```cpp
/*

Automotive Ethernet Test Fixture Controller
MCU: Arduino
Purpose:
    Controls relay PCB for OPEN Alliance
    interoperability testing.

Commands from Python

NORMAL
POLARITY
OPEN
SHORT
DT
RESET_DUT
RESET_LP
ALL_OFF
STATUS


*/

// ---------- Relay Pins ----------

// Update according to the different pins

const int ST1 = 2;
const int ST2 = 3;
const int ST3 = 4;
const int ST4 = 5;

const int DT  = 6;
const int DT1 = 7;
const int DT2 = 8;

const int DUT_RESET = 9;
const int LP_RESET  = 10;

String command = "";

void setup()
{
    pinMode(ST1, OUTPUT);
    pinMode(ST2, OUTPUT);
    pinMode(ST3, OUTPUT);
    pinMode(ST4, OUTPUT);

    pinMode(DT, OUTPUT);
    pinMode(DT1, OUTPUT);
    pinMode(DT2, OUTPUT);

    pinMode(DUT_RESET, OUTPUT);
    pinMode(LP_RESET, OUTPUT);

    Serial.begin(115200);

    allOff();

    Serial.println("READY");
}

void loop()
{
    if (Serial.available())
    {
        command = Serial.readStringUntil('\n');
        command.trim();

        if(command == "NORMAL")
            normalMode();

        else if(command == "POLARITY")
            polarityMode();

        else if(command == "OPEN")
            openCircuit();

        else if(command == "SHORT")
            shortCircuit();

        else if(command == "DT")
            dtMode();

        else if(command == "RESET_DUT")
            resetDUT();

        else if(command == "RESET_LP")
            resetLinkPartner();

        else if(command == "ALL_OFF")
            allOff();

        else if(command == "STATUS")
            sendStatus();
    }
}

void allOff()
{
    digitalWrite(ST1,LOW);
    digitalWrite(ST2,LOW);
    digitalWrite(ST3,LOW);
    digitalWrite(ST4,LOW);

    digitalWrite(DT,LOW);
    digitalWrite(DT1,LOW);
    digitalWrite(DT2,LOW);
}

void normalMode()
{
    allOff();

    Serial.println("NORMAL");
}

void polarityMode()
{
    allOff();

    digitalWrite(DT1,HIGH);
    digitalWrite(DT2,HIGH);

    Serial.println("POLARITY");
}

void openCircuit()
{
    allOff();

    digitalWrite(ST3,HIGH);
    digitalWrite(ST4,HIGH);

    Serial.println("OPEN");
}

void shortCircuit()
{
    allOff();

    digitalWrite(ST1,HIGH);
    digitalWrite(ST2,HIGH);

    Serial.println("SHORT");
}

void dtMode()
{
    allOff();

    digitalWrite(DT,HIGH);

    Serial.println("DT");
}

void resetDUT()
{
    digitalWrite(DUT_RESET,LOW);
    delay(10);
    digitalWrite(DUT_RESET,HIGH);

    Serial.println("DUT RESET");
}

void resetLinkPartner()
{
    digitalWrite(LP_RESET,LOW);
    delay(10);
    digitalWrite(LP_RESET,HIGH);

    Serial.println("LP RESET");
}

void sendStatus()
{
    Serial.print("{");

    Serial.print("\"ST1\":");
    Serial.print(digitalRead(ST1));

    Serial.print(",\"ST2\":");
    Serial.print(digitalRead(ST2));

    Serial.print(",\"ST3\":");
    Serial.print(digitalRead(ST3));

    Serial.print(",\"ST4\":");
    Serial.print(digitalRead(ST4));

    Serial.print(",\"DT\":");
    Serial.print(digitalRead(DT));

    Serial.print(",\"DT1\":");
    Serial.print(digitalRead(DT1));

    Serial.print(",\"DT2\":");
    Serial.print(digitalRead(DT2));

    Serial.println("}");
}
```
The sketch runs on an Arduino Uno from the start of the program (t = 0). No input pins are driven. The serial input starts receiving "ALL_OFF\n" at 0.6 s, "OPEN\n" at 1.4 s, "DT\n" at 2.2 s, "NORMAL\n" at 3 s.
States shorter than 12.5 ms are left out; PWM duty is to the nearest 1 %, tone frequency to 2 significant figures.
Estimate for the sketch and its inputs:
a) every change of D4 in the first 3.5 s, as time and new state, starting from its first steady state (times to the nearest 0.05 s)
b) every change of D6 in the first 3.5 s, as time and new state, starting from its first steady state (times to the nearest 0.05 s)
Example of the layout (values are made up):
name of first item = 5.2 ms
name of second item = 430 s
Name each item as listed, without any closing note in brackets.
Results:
every change of D4 in the first 3.5 s, as time and new state, starting from its first steady state = 0 s low; 1.4 s high; 2.2 s low
every change of D6 in the first 3.5 s, as time and new state, starting from its first steady state = 0 s low; 2.2 s high; 3 s low
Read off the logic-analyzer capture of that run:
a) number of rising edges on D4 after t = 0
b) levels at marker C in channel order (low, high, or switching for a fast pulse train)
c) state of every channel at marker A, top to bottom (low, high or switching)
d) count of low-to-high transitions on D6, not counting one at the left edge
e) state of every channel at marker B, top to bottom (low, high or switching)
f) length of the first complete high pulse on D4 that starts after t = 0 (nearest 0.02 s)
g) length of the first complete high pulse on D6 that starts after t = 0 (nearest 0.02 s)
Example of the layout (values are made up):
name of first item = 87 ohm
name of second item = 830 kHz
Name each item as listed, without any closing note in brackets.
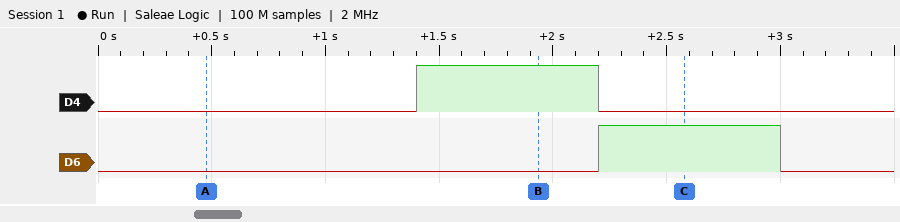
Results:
number of rising edges on D4 after t = 0 = 1
levels at marker C in channel order = D4 low, D6 high
state of every channel at marker A, top to bottom = D4 low, D6 low
count of low-to-high transitions on D6, not counting one at the left edge = 1
state of every channel at marker B, top to bottom = D4 high, D6 low
length of the first complete high pulse on D4 that starts after t = 0 = 0.80 s
length of the first complete high pulse on D6 that starts after t = 0 = 0.80 s
